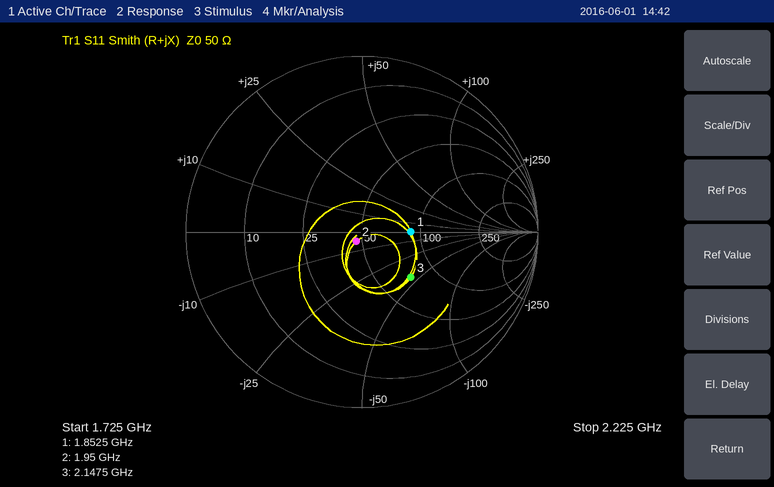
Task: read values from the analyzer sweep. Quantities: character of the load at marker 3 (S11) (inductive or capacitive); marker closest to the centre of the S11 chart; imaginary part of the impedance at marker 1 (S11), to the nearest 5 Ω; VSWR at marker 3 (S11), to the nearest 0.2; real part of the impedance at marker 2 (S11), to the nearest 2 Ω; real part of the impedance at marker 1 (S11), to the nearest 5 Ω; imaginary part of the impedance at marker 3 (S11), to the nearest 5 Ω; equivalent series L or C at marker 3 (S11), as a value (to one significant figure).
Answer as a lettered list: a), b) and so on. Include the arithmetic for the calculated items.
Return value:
a) capacitive
b) marker 2
c) 0 Ω
d) 2.2
e) 46 Ω
f) 90 Ω
g) -45 Ω
h) C = 1/(2π × 2.1475 GHz × 45 Ω) ≈ 2 pF
